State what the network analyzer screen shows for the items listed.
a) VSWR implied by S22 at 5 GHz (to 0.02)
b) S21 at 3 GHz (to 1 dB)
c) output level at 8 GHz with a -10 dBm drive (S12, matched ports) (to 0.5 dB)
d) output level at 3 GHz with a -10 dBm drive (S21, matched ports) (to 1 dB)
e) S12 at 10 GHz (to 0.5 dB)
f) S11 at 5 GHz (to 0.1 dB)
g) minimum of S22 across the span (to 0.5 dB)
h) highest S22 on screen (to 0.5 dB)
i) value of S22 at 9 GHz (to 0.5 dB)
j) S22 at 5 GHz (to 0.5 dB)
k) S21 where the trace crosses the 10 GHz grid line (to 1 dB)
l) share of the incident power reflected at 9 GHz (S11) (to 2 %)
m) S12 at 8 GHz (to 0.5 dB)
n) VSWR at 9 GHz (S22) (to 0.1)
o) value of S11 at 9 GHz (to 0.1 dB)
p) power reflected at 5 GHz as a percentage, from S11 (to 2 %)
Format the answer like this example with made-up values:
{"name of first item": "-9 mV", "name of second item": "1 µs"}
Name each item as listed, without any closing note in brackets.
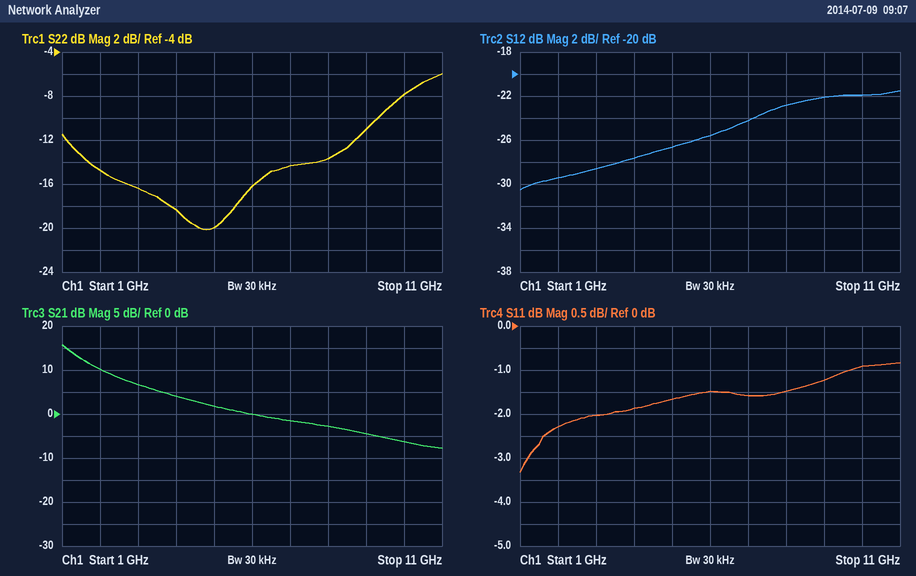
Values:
{"VSWR implied by S22 at 5 GHz": "1.22", "S21 at 3 GHz": "7 dB", "output level at 8 GHz with a -10 dBm drive (S12, matched ports)": "-33.0 dBm", "output level at 3 GHz with a -10 dBm drive (S21, matched ports)": "-3 dBm", "S12 at 10 GHz": "-22.0 dB", "S11 at 5 GHz": "-1.7 dB", "minimum of S22 across the span": "-20.0 dB", "highest S22 on screen": "-6.0 dB", "value of S22 at 9 GHz": "-11.0 dB", "S22 at 5 GHz": "-20.0 dB", "S21 where the trace crosses the 10 GHz grid line": "-6 dB", "share of the incident power reflected at 9 GHz (S11)": "76 %", "S12 at 8 GHz": "-23.0 dB", "VSWR at 9 GHz (S22)": "1.8", "value of S11 at 9 GHz": "-1.2 dB", "power reflected at 5 GHz as a percentage, from S11": "68 %"}
